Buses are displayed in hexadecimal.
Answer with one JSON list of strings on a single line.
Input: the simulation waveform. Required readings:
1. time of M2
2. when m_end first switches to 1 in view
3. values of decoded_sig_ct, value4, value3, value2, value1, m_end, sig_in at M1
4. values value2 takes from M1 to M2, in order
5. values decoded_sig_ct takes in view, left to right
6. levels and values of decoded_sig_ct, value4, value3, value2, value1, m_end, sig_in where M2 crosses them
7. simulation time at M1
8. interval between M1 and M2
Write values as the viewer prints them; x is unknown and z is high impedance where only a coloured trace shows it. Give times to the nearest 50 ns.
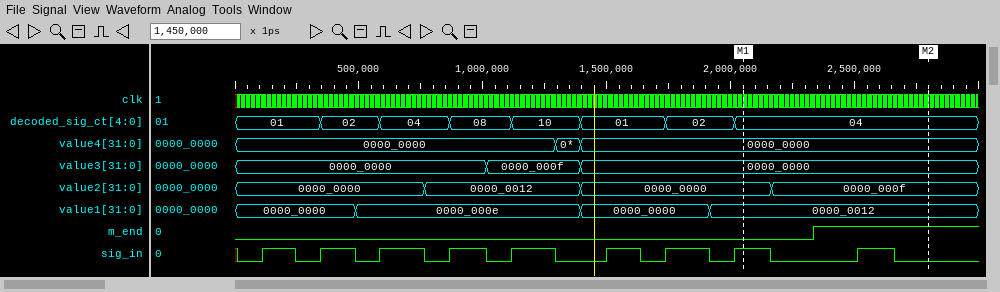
["2800 ns", "2350 ns", "decoded_sig_ct=04, value4=0000_0000, value3=0000_0000, value2=0000_0000, value1=0000_0012, m_end=0, sig_in=1", "0000_0000, 0000_000f", "01, 02, 04, 08, 10, 01, 02, 04", "decoded_sig_ct=04, value4=0000_0000, value3=0000_0000, value2=0000_000f, value1=0000_0012, m_end=1, sig_in=0", "2050 ns", "750 ns"]
